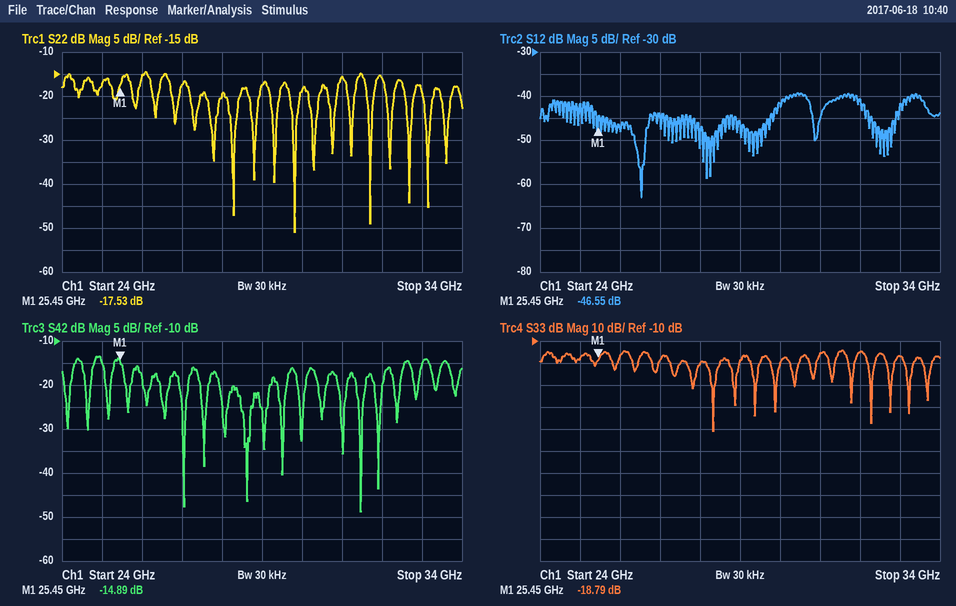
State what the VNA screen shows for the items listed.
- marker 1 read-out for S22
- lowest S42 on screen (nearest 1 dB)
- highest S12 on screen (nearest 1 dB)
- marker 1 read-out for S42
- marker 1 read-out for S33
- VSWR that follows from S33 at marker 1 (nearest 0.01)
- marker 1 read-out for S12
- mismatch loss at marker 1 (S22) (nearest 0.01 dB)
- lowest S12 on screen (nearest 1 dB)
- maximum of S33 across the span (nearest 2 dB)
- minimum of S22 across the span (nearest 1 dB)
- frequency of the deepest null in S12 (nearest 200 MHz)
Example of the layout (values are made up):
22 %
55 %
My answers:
-17.53 dB
-49 dB
-39 dB
-14.89 dB
-18.79 dB
1.26
-46.55 dB
0.08 dB
-63 dB
-14 dB
-51 dB
26.6 GHz
